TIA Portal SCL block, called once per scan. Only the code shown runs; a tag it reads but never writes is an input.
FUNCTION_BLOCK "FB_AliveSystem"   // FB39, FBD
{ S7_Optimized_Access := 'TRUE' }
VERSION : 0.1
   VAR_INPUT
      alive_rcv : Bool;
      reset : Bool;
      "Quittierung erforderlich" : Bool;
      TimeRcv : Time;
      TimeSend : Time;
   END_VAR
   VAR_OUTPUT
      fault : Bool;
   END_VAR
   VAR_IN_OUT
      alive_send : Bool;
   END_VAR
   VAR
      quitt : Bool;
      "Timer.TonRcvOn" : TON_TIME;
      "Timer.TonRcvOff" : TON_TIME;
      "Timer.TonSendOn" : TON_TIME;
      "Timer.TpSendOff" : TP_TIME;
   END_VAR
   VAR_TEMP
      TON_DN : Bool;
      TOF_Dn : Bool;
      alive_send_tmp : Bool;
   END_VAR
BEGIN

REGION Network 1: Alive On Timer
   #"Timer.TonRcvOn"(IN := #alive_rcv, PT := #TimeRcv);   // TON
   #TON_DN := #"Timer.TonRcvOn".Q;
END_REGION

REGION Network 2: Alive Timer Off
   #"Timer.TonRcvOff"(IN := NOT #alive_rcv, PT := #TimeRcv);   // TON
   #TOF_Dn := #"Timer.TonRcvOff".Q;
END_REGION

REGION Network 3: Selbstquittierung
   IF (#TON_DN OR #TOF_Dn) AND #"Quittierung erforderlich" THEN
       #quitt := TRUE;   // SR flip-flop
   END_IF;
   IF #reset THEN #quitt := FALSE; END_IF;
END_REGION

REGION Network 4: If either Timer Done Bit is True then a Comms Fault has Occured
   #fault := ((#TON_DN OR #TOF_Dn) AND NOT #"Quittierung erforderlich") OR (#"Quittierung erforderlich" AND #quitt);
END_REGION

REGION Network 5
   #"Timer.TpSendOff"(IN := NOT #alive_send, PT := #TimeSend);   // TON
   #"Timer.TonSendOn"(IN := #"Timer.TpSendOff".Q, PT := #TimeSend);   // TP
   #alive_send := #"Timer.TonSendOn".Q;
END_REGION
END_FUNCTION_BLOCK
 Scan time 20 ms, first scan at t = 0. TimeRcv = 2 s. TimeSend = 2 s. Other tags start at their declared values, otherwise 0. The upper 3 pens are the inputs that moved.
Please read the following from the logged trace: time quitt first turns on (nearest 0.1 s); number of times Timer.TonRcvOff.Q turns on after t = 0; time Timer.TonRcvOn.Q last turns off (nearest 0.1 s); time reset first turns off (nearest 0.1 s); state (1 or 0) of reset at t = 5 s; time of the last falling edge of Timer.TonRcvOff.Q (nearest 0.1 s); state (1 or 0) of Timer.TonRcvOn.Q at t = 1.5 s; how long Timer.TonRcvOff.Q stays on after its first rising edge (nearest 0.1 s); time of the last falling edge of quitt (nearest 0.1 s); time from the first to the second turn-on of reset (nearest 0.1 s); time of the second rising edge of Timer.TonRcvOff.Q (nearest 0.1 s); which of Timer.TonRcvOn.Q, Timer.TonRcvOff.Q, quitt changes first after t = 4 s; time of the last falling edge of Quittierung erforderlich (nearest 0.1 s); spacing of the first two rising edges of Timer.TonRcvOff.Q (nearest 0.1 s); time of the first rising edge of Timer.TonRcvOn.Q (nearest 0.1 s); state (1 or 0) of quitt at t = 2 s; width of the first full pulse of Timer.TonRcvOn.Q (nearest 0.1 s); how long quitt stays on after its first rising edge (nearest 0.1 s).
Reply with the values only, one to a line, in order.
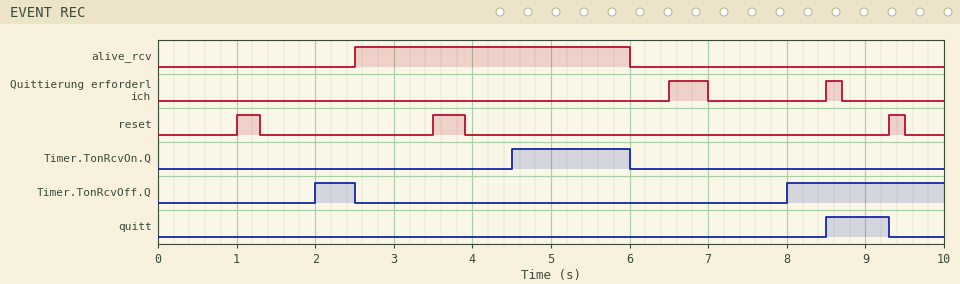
8.5 s
2
6.0 s
1.3 s
0
2.5 s
0
0.5 s
9.3 s
2.5 s
8.0 s
Timer.TonRcvOn.Q
8.7 s
6.0 s
4.5 s
0
1.5 s
0.8 s
